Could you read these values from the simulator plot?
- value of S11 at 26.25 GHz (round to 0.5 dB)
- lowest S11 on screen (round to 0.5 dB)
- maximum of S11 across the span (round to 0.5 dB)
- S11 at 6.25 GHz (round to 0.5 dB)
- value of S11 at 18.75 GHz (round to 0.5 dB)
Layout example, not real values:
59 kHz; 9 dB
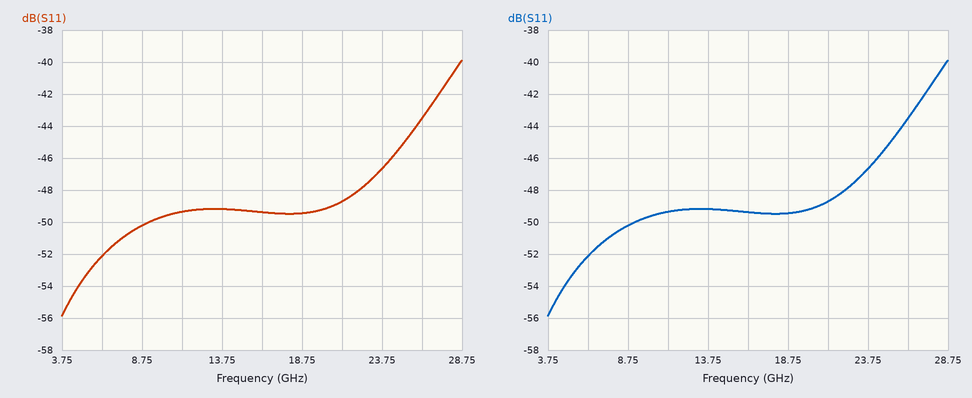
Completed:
-43.5 dB; -56.0 dB; -40.0 dB; -52.0 dB; -49.5 dB
